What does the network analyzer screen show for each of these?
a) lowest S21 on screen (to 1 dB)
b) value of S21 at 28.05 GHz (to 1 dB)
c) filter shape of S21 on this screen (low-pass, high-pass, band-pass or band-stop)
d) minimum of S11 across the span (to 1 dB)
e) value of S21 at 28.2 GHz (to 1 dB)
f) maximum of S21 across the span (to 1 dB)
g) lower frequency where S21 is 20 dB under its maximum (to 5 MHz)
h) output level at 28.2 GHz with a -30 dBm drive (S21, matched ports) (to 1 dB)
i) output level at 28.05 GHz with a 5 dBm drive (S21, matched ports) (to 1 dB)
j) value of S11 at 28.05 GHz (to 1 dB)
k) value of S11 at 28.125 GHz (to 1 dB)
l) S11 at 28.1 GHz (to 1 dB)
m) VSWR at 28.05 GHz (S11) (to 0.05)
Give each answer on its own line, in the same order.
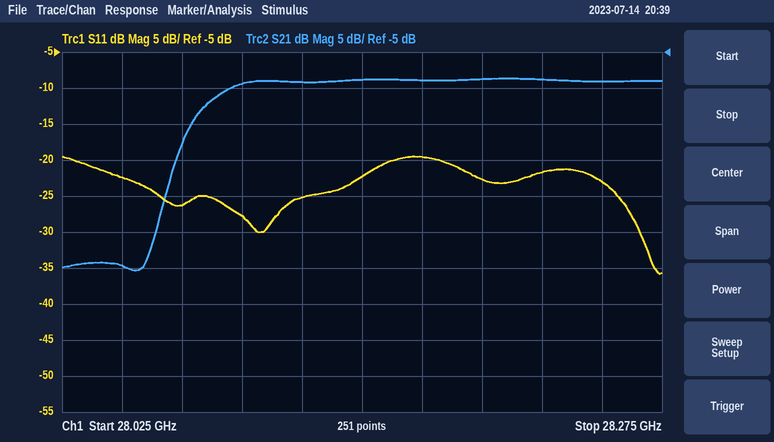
-35 dB
-35 dB
high-pass
-36 dB
-9 dB
-9 dB
28.065 GHz
-39 dBm
-30 dBm
-22 dB
-25 dB
-28 dB
1.15
